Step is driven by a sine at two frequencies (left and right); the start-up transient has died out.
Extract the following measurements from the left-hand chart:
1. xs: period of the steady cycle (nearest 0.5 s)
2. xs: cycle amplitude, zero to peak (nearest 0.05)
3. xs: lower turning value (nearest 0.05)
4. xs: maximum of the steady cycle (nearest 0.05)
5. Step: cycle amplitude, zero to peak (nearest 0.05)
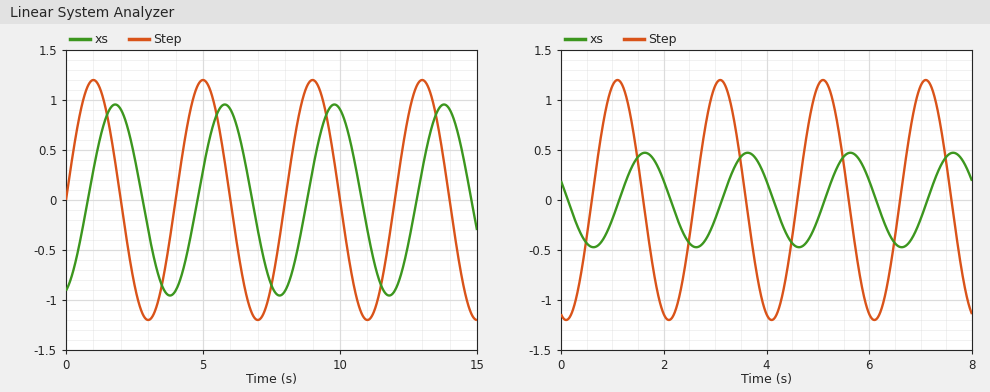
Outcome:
4.0 s
0.95
-0.95
0.95
1.20
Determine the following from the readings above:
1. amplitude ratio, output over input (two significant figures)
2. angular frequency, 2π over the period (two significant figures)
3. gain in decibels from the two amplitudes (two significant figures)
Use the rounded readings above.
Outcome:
0.79
1.6 rad/s
-2.0 dB
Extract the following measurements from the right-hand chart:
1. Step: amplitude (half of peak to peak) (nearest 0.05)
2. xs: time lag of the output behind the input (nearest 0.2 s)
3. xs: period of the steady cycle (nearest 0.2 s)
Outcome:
1.20
0.6 s
2.0 s
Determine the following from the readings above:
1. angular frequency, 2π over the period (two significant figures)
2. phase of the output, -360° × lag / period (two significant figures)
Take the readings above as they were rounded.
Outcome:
3.1 rad/s
-110°
